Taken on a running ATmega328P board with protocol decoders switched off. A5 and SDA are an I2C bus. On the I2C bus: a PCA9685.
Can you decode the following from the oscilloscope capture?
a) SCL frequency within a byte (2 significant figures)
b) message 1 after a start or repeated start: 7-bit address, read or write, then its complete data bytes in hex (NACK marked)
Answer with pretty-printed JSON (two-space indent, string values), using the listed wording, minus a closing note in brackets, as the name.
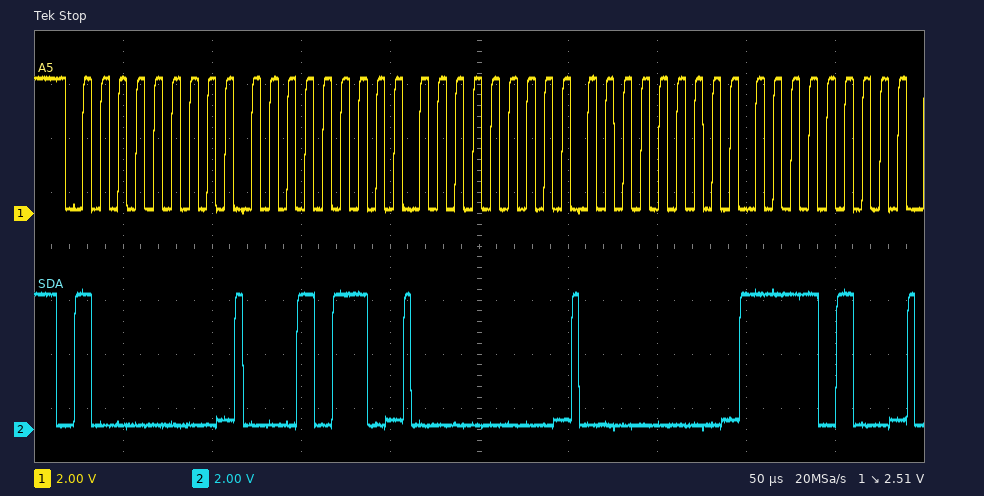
{
  "SCL frequency within a byte": "100 kHz",
  "message 1 after a start or repeated start: 7-bit address, read or write, then its complete data bytes in hex": "0x40 write: 16 00 00 F4"
}
